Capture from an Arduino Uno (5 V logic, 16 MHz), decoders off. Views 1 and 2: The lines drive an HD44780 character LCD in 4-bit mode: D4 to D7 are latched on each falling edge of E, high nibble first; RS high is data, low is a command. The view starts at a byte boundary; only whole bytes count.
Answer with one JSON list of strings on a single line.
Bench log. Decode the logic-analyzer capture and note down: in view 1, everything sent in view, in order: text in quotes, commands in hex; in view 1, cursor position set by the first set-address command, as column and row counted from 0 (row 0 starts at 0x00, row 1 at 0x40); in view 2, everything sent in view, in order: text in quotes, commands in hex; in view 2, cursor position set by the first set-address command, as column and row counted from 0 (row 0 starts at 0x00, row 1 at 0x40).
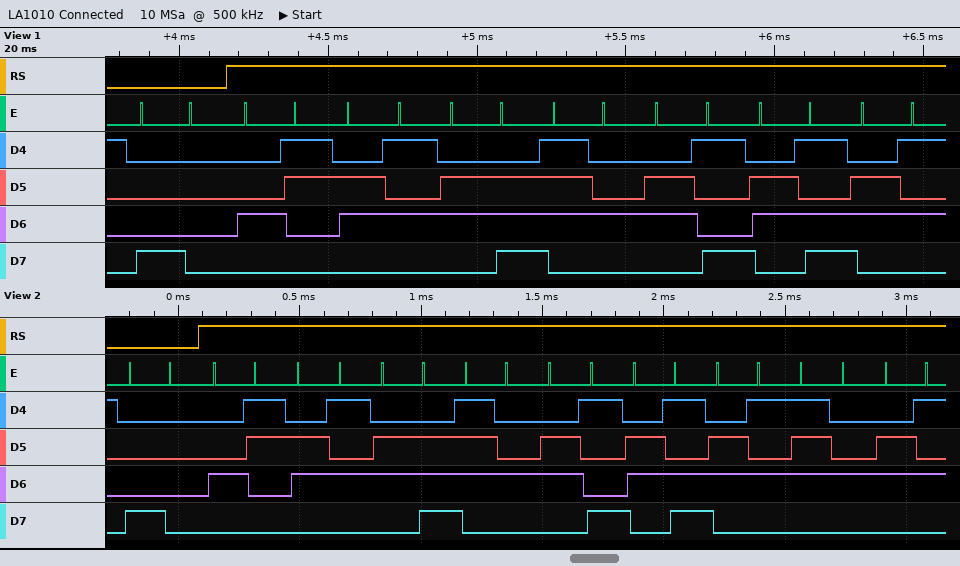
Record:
["0x80 \"Centime\"", "column 0, row 0", "0x80 \"Centimete\"", "column 0, row 0"]
